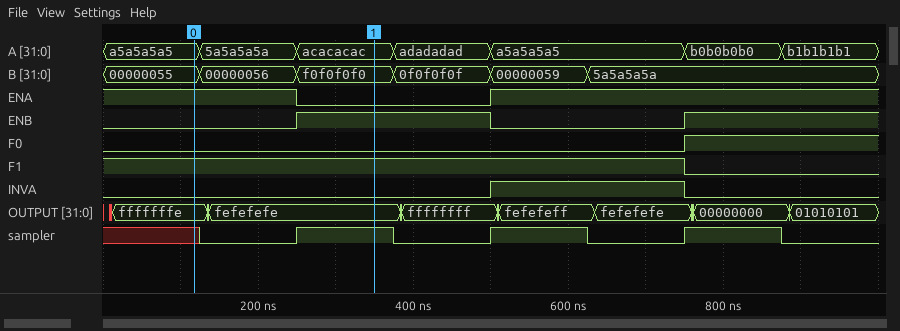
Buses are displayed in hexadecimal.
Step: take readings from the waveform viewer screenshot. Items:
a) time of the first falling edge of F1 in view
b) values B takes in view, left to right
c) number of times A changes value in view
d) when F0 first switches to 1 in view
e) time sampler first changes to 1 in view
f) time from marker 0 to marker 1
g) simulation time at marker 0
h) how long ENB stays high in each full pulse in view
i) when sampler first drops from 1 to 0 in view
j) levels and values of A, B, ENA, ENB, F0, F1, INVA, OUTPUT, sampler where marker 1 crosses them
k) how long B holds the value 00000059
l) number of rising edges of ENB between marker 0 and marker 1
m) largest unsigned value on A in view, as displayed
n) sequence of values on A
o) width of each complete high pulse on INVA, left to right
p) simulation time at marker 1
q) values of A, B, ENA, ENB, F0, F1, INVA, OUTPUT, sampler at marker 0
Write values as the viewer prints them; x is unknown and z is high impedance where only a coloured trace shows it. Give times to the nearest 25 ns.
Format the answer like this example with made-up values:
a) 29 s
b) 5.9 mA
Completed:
a) 750 ns
b) 00000055, 00000056, f0f0f0f0, 0f0f0f0f, 00000059, 5a5a5a5a
c) 6
d) 750 ns
e) 250 ns
f) 225 ns
g) 125 ns
h) 250 ns
i) 375 ns
j) A=acacacac, B=f0f0f0f0, ENA=0, ENB=1, F0=0, F1=1, INVA=0, OUTPUT=fefefefe, sampler=1
k) 125 ns
l) 1
m) b1b1b1b1
n) a5a5a5a5, 5a5a5a5a, acacacac, adadadad, a5a5a5a5, b0b0b0b0, b1b1b1b1
o) 250 ns
p) 350 ns
q) A=a5a5a5a5, B=00000055, ENA=1, ENB=0, F0=0, F1=1, INVA=0, OUTPUT=fffffffe, sampler=x
